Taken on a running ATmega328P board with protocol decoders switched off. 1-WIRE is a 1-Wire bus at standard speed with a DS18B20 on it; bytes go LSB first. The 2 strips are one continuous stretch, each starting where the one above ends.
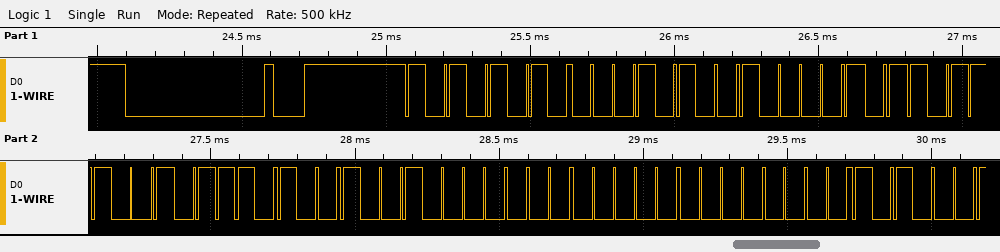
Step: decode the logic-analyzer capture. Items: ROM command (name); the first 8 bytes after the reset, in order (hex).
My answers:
Match ROM
55 28 A1 9D 2E 09 00 00
